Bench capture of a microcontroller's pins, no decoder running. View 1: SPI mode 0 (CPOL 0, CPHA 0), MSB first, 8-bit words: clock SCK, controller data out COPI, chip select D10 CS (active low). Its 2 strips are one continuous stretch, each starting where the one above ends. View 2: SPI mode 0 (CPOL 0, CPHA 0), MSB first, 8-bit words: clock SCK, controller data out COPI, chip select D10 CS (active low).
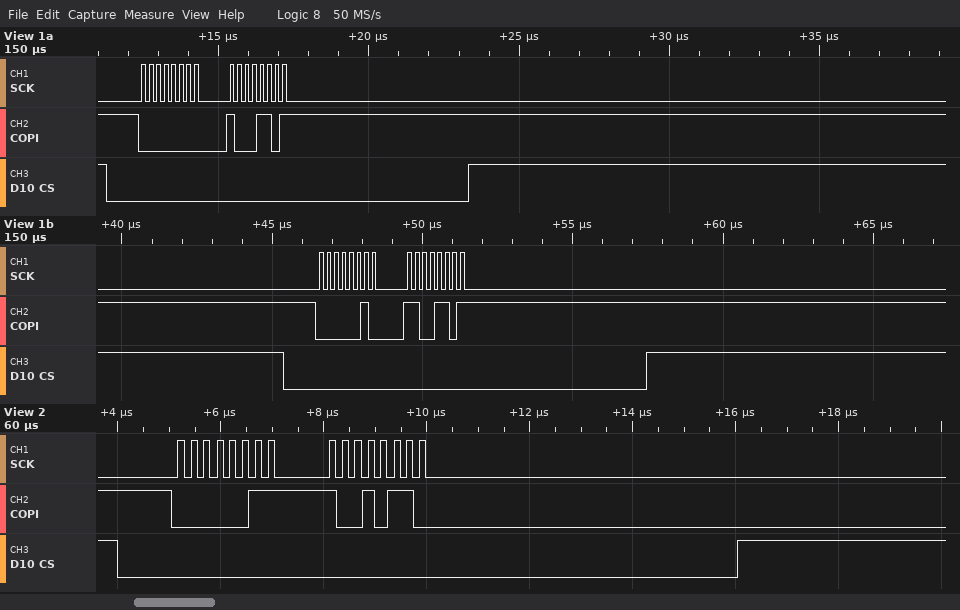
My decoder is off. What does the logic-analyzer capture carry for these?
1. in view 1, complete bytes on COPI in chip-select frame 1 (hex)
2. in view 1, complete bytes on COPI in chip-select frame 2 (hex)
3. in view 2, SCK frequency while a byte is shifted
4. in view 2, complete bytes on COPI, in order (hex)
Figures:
00 8D
02 CD
4 MHz
03 96
